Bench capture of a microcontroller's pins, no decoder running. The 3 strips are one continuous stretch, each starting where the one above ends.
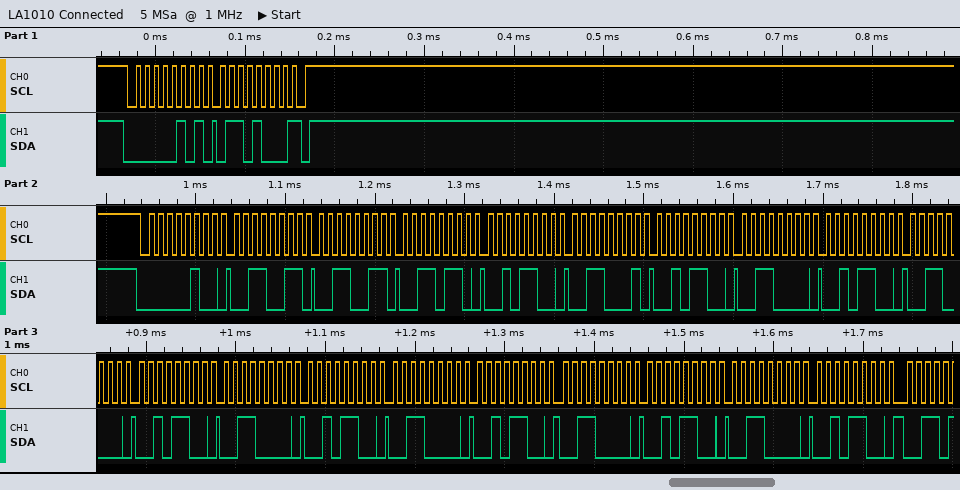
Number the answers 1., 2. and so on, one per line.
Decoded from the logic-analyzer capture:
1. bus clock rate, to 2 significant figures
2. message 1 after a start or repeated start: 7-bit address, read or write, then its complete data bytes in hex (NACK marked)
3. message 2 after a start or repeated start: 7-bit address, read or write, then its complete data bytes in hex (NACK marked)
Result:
1. 100 kHz
2. 0x02 read: 68 NACK
3. 0x02 write: 33 33 36 2C 31 2C 30 2C 30 2C 30 2C 30 2C 30 2C 30 2C
